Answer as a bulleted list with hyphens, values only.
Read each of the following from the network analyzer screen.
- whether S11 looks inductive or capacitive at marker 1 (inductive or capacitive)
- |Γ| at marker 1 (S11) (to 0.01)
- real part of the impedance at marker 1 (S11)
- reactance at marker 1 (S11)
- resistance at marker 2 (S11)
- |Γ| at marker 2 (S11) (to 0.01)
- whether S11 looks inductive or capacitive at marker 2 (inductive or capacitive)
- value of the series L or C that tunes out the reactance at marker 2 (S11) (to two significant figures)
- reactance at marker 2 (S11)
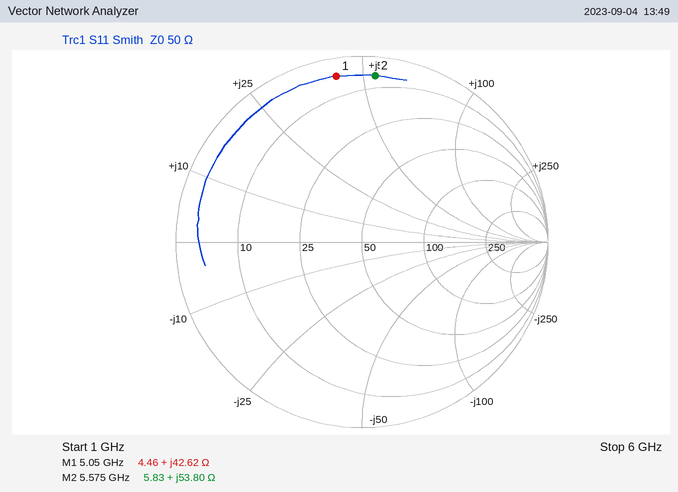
- inductive
- 0.90
- 4.46 Ω
- +42.62 Ω
- 5.83 Ω
- 0.90
- inductive
- 530 fF
- +53.80 Ω
